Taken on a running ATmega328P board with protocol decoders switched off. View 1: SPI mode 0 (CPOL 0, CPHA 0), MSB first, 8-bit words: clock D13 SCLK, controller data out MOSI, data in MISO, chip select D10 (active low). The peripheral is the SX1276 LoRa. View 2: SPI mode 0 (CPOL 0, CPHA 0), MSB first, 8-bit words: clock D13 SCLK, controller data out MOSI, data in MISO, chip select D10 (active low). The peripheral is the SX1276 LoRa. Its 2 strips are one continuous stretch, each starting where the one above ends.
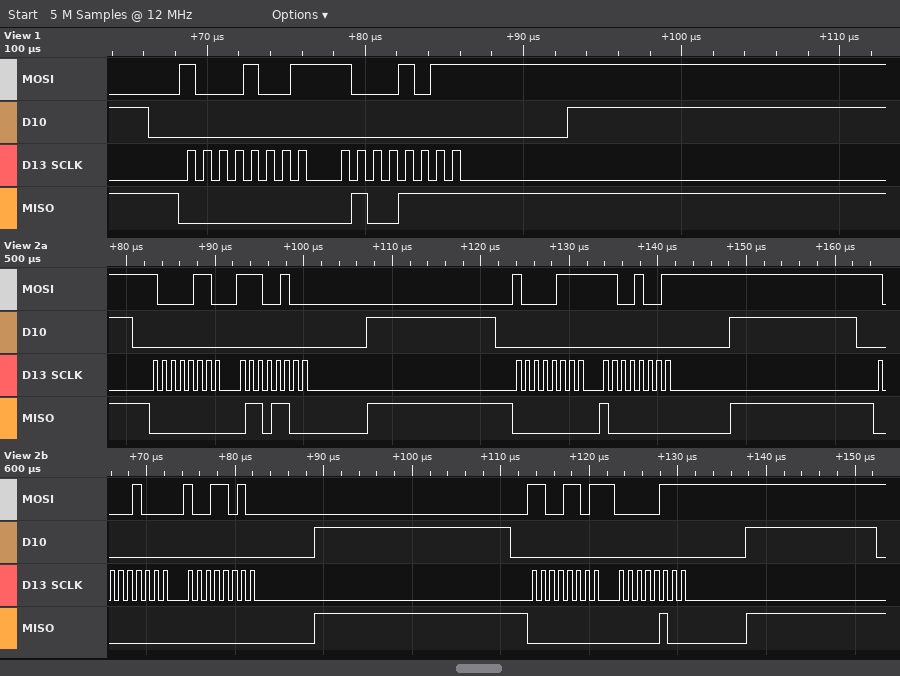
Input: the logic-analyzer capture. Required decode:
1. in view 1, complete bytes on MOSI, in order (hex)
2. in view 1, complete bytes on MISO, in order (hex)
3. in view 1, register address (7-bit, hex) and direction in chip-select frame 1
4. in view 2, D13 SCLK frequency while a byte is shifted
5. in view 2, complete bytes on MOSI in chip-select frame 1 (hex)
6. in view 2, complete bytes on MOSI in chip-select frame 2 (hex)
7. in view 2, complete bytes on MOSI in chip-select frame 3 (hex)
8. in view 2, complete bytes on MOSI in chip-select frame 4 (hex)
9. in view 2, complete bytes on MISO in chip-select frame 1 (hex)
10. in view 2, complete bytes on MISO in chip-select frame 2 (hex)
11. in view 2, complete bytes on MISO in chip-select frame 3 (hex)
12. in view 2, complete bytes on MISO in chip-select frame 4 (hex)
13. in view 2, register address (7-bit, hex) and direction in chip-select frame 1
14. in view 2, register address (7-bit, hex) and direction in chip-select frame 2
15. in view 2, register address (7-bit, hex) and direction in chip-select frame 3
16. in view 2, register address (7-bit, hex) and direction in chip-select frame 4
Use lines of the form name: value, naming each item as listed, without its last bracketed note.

in view 1, complete bytes on MOSI, in order: 0x89 0x8B
in view 1, complete bytes on MISO, in order: 0x00 0x4F
in view 1, register address (7-bit, hex) and direction in chip-select frame 1: 0x09 write
in view 2, D13 SCLK frequency while a byte is shifted: 1 MHz
in view 2, complete bytes on MOSI in chip-select frame 1: 86 E4
in view 2, complete bytes on MOSI in chip-select frame 2: 87 C9
in view 2, complete bytes on MOSI in chip-select frame 3: 88 9A
in view 2, complete bytes on MOSI in chip-select frame 4: CD 07
in view 2, complete bytes on MISO in chip-select frame 1: 00 6C
in view 2, complete bytes on MISO in chip-select frame 2: 00 80
in view 2, complete bytes on MISO in chip-select frame 3: 00 00
in view 2, complete bytes on MISO in chip-select frame 4: 00 04
in view 2, register address (7-bit, hex) and direction in chip-select frame 1: 0x06 write
in view 2, register address (7-bit, hex) and direction in chip-select frame 2: 0x07 write
in view 2, register address (7-bit, hex) and direction in chip-select frame 3: 0x08 write
in view 2, register address (7-bit, hex) and direction in chip-select frame 4: 0x4D write
